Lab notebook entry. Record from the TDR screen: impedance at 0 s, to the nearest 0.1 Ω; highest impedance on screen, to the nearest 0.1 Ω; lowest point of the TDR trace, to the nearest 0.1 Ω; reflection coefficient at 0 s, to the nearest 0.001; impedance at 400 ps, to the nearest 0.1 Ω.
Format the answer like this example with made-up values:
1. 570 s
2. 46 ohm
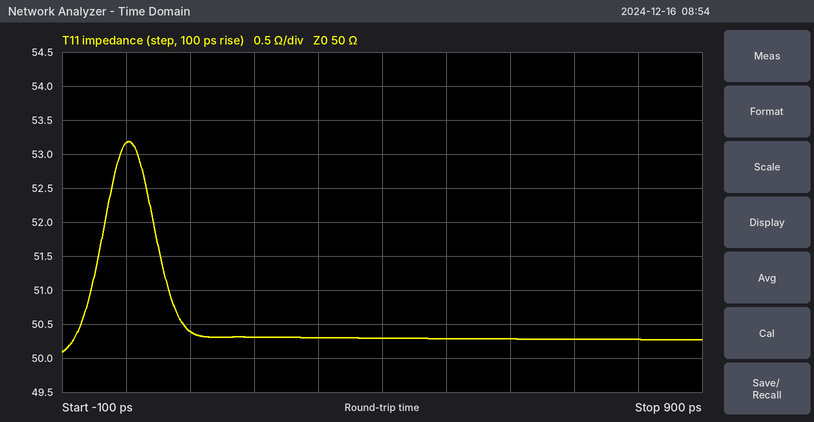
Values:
1. 53.2 Ω
2. 53.2 Ω
3. 50.1 Ω
4. +0.031
5. 50.3 Ω
